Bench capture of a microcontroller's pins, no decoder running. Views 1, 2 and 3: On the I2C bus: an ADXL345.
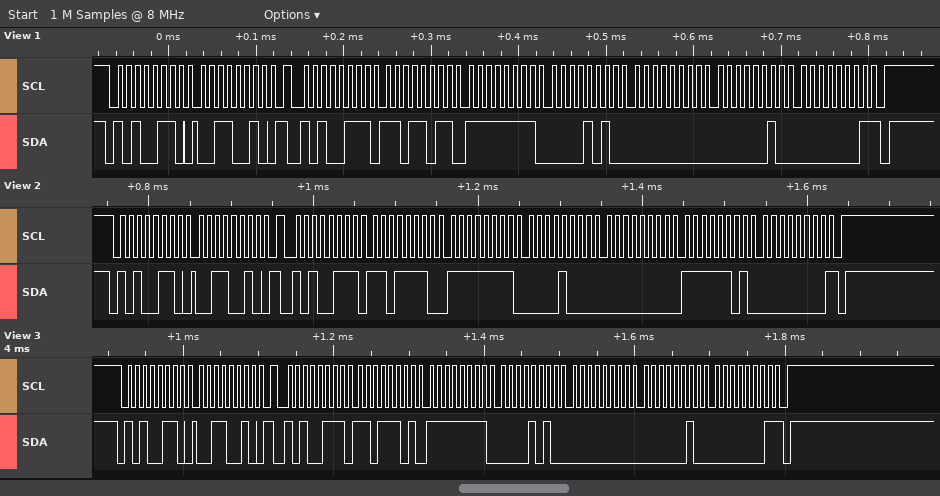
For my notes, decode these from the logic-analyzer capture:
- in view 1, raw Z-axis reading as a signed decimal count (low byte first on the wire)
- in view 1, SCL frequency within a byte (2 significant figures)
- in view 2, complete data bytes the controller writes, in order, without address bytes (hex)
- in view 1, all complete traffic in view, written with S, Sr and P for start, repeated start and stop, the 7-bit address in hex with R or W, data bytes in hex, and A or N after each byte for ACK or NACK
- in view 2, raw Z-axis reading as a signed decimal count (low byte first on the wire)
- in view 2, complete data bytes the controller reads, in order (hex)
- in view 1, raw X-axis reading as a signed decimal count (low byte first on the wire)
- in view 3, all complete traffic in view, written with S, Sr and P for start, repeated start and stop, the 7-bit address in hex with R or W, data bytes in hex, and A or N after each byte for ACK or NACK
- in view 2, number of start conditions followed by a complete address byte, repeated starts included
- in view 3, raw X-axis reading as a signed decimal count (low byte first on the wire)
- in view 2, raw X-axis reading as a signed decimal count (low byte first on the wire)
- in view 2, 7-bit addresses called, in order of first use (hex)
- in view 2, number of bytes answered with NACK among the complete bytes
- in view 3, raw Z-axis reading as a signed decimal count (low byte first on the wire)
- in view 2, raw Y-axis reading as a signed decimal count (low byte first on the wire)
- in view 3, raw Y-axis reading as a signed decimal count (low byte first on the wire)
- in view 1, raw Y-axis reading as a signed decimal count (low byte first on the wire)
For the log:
258
100 kHz
32
S 53W A 32 A Sr 53R A DB A FF A 0A A 00 A 02 A 01 N P
253
DE FF 08 00 FD 00
-37
S 53W A 32 A Sr 53R A DD A FF A 0A A 00 A 02 A 01 N P
2
-35
-34
0x53
1
258
8
10
10
